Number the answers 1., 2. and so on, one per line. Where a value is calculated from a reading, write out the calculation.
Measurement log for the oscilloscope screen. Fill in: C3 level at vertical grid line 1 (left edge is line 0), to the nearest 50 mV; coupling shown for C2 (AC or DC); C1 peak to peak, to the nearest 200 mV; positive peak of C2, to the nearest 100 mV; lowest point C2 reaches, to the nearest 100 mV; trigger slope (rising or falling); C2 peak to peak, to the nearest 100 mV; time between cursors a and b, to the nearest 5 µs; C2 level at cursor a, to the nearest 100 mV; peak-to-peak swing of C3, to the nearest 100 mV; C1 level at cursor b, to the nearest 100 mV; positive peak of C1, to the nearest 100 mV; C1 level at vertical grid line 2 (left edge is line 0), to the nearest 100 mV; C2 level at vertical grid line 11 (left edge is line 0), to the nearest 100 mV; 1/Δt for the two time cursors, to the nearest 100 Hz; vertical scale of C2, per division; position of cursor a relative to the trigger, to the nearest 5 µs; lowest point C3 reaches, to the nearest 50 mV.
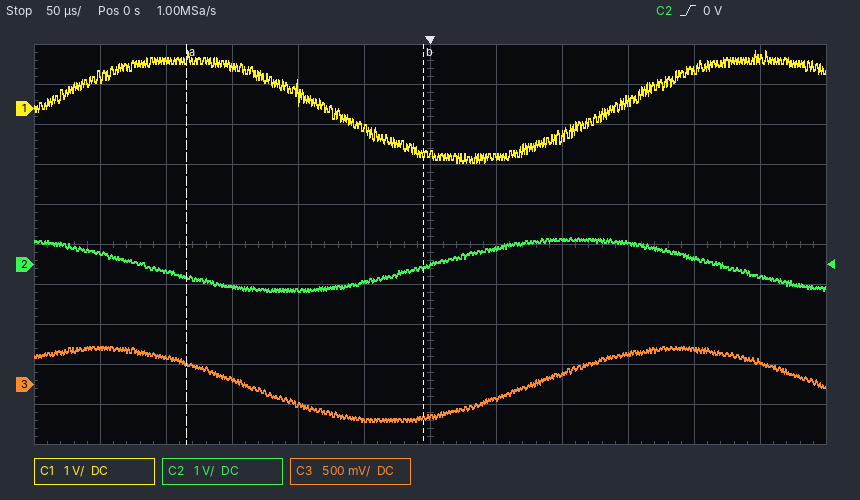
1. 450 mV
2. DC
3. 2.8 V
4. 700 mV
5. -700 mV
6. rising
7. 700 mV − (-700 mV) = 1.4 V
8. 180 µs
9. -300 mV
10. 900 mV
11. -1.1 V
12. 1.4 V
13. 1.2 V
14. -300 mV
15. 1 / 180 µs ≈ 5.6 kHz
16. 1 V
17. -185 µs
18. -450 mV
